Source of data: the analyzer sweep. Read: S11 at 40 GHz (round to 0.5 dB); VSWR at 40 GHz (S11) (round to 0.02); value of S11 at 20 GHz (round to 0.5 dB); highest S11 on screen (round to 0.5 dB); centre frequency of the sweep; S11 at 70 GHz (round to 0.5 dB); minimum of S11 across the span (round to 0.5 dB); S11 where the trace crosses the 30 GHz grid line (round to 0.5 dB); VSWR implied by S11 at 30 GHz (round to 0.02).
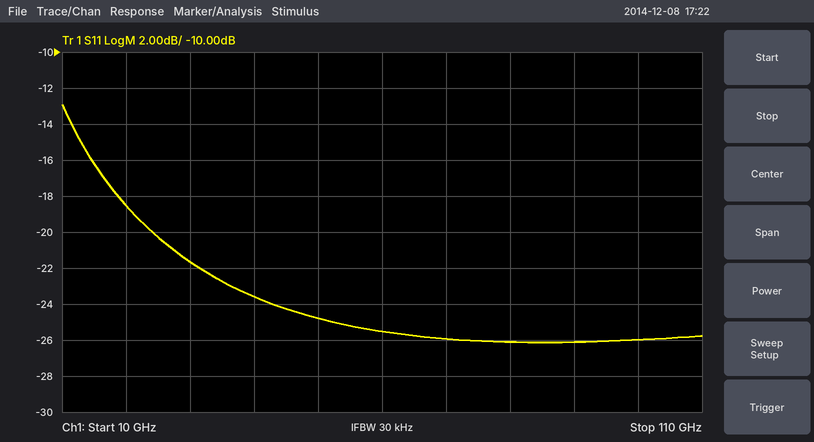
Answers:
-23.5 dB
1.14
-18.5 dB
-13.0 dB
60 GHz
-26.0 dB
-26.0 dB
-21.5 dB
1.18
